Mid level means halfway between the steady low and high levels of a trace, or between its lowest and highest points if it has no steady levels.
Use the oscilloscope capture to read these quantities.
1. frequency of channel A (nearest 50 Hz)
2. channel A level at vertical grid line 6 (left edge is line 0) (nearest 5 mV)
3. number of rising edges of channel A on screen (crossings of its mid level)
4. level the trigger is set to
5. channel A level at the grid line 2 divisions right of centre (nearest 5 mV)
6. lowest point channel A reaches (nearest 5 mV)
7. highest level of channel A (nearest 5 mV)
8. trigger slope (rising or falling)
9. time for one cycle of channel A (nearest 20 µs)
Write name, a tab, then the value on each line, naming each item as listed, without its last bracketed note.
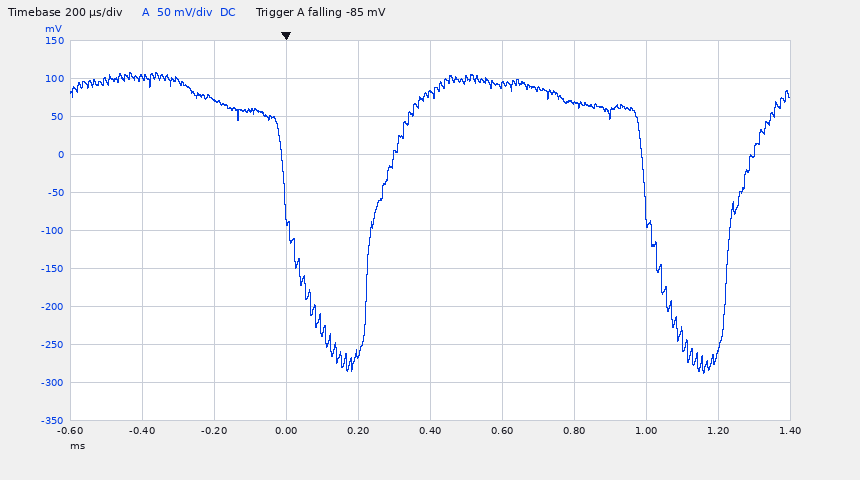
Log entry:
frequency of channel A	1.00 kHz
channel A level at vertical grid line 6 (left edge is line 0)	90 mV
number of rising edges of channel A on screen	2
level the trigger is set to	-85 mV
channel A level at the grid line 2 divisions right of centre	70 mV
lowest point channel A reaches	-290 mV
highest level of channel A	110 mV
trigger slope	falling
time for one cycle of channel A	1.00 ms
